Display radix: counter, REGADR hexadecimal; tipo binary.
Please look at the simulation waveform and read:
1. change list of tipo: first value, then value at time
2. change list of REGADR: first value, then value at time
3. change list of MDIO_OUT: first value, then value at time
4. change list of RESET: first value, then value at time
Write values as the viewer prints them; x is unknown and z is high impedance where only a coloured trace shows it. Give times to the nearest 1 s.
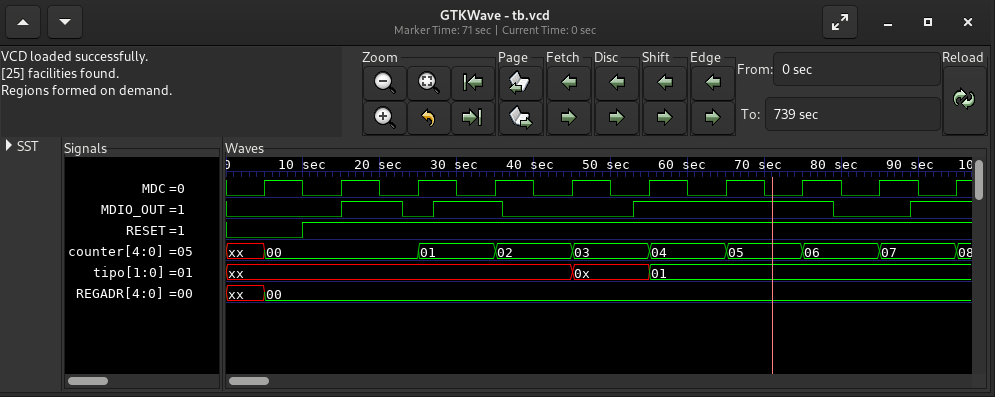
xx, 0x at 45 s, 01 at 55 s
xx, 00 at 5 s
0, 1 at 15 s, 0 at 23 s, 1 at 27 s, 0 at 36 s, 1 at 53 s, 0 at 79 s, 1 at 89 s
0, 1 at 10 s
